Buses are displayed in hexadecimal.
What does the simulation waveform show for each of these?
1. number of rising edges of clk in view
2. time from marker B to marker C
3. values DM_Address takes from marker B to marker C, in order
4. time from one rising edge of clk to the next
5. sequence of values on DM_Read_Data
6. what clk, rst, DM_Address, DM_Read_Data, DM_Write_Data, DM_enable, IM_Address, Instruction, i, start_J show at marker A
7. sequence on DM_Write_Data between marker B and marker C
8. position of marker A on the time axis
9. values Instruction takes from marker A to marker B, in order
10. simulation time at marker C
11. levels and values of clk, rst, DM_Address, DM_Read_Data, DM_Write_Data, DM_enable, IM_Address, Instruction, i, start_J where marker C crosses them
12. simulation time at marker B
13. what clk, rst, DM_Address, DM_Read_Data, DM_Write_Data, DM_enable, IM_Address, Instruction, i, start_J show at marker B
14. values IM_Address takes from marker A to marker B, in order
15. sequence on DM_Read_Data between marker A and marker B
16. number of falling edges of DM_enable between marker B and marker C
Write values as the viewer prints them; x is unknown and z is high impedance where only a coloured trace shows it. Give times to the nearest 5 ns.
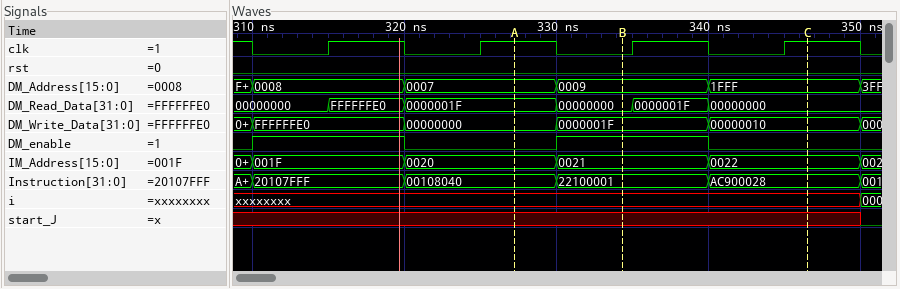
4
10 ns
0009, 1FFF
10 ns
00000000, FFFFFFE0, 0000001F, 00000000, 0000001F, 00000000
clk=1, rst=0, DM_Address=0007, DM_Read_Data=0000001F, DM_Write_Data=00000000, DM_enable=0, IM_Address=0020, Instruction=00108040, i=xxxxxxxx, start_J=x
0000001F, 00000010
325 ns
00108040, 22100001
345 ns
clk=1, rst=0, DM_Address=1FFF, DM_Read_Data=00000000, DM_Write_Data=00000010, DM_enable=0, IM_Address=0022, Instruction=AC900028, i=xxxxxxxx, start_J=x
335 ns
clk=0, rst=0, DM_Address=0009, DM_Read_Data=00000000, DM_Write_Data=0000001F, DM_enable=1, IM_Address=0021, Instruction=22100001, i=xxxxxxxx, start_J=x
0020, 0021
0000001F, 00000000
1
